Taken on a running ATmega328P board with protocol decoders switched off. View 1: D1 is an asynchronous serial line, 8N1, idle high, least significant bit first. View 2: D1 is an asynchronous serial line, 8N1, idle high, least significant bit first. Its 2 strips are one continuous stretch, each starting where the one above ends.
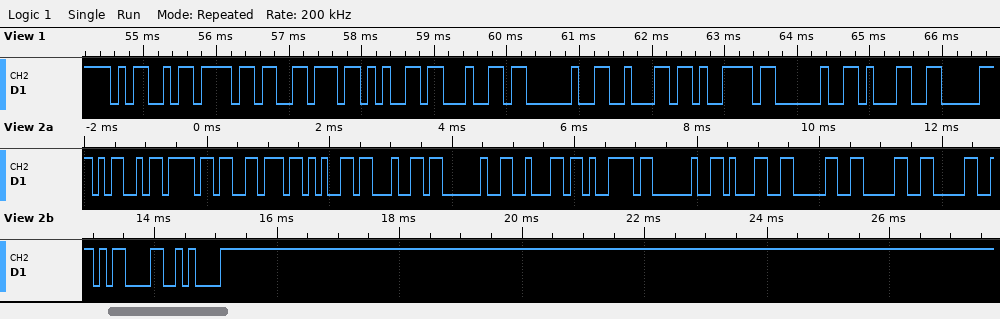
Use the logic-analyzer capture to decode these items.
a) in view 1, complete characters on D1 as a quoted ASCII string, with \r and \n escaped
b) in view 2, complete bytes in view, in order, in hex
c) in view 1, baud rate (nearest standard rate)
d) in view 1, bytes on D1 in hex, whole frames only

"Moved by 1"
0x4D 0x6F 0x76 0x65 0x64 0x20 0x62 0x79 0x20 0x31 0x30 0x30 0x30 0x0D 0x0A
9600 baud
0x4D 0x6F 0x76 0x65 0x64 0x20 0x62 0x79 0x20 0x31
